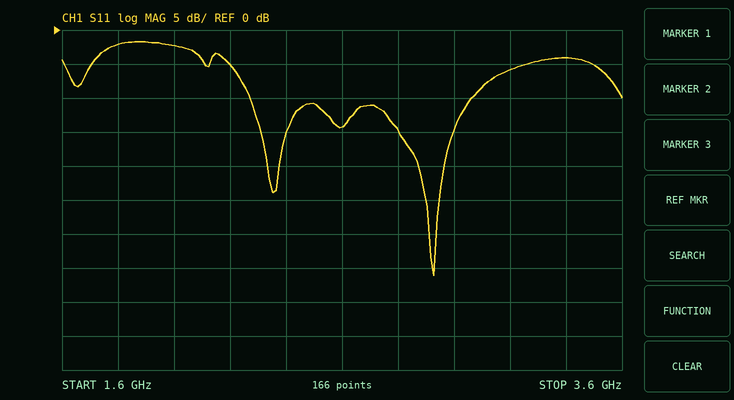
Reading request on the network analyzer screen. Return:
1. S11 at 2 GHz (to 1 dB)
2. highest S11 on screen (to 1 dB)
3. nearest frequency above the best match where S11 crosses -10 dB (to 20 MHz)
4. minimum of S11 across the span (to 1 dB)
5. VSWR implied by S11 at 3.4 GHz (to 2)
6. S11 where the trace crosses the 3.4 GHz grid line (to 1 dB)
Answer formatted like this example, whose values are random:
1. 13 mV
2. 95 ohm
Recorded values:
1. -2 dB
2. -2 dB
3. 3.06 GHz
4. -36 dB
5. 4
6. -4 dB
